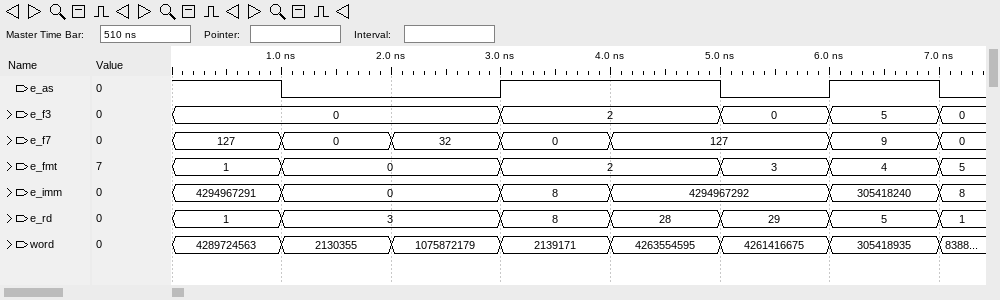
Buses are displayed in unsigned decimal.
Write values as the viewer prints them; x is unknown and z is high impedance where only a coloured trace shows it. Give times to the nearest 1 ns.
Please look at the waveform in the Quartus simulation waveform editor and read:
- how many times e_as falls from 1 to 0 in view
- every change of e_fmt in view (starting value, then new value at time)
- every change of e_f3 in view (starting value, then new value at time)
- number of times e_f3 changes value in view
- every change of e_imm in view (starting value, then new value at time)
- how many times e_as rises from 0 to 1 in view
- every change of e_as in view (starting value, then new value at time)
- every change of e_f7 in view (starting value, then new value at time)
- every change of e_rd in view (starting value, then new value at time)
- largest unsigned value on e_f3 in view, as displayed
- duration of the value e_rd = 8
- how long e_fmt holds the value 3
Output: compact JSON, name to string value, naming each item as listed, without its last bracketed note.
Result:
{"how many times e_as falls from 1 to 0 in view": "3", "every change of e_fmt in view": "1, 0 at 1 ns, 2 at 3 ns, 3 at 5 ns, 4 at 6 ns, 5 at 7 ns", "every change of e_f3 in view": "0, 2 at 3 ns, 0 at 5 ns, 5 at 6 ns, 0 at 7 ns", "number of times e_f3 changes value in view": "4", "every change of e_imm in view": "4294967291, 0 at 1 ns, 8 at 3 ns, 4294967292 at 4 ns, 305418240 at 6 ns, 8 at 7 ns", "how many times e_as rises from 0 to 1 in view": "2", "every change of e_as in view": "1, 0 at 1 ns, 1 at 3 ns, 0 at 5 ns, 1 at 6 ns, 0 at 7 ns", "every change of e_f7 in view": "127, 0 at 1 ns, 32 at 2 ns, 0 at 3 ns, 127 at 4 ns, 9 at 6 ns, 0 at 7 ns", "every change of e_rd in view": "1, 3 at 1 ns, 8 at 3 ns, 28 at 4 ns, 29 at 5 ns, 5 at 6 ns, 1 at 7 ns", "largest unsigned value on e_f3 in view, as displayed": "5", "duration of the value e_rd = 8": "1 ns", "how long e_fmt holds the value 3": "1 ns"}
